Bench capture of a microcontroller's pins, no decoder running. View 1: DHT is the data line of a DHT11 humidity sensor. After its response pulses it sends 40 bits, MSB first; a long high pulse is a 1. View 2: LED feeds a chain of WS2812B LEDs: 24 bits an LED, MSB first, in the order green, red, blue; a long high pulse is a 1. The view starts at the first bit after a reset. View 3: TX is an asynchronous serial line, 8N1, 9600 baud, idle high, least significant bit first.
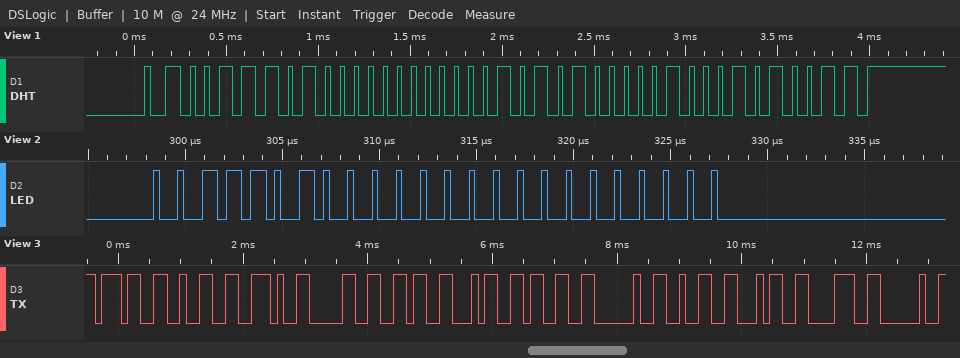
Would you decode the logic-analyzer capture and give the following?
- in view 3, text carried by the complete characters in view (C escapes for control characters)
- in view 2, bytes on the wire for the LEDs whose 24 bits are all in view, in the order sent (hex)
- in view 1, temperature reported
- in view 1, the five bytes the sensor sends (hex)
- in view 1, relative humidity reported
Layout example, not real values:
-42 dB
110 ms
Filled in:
"72.0643 248 "
3A 00 00
21.4 °C
3A 00 15 04 53
58 %
